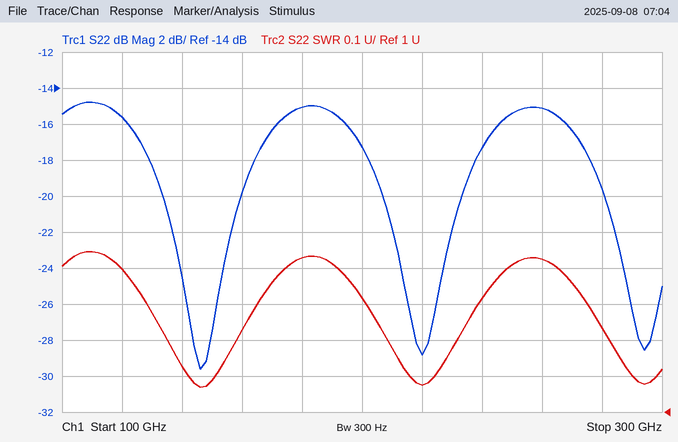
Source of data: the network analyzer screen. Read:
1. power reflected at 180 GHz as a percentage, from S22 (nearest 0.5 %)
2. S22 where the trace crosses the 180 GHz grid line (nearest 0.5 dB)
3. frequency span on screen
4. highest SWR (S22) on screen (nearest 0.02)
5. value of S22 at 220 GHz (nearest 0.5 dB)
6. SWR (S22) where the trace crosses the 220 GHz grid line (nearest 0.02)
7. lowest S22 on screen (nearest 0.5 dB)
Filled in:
3.0 %
-15.0 dB
200 GHz
1.44
-29.0 dB
1.08
-29.5 dB
